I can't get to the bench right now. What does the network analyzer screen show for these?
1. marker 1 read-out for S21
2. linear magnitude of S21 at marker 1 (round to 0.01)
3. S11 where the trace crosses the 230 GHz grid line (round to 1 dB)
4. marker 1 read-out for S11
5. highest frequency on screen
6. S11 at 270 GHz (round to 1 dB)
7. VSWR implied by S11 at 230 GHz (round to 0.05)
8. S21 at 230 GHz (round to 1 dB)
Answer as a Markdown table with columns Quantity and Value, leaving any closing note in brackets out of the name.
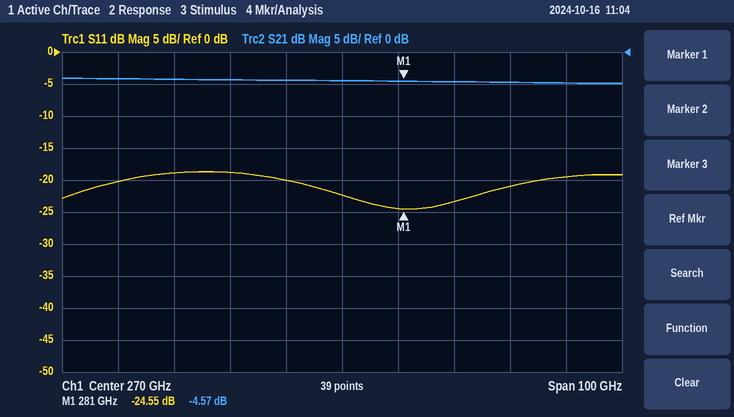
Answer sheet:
| Quantity | Value |
|---|---|
| marker 1 read-out for S21 | -4.57 dB |
| linear magnitude of S21 at marker 1 | 0.59 |
| S11 where the trace crosses the 230 GHz grid line | -20 dB |
| marker 1 read-out for S11 | -24.55 dB |
| highest frequency on screen | 320 GHz |
| S11 at 270 GHz | -22 dB |
| VSWR implied by S11 at 230 GHz | 1.20 |
| S21 at 230 GHz | -4 dB |
